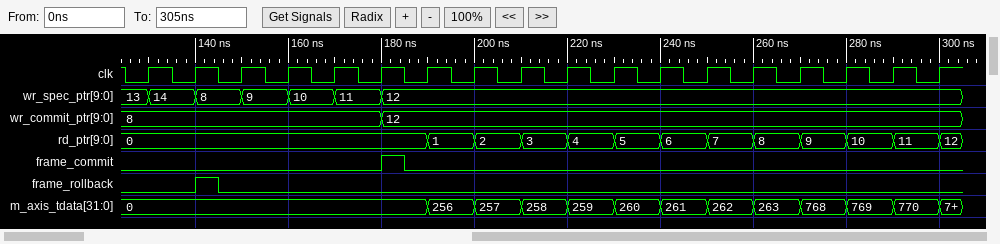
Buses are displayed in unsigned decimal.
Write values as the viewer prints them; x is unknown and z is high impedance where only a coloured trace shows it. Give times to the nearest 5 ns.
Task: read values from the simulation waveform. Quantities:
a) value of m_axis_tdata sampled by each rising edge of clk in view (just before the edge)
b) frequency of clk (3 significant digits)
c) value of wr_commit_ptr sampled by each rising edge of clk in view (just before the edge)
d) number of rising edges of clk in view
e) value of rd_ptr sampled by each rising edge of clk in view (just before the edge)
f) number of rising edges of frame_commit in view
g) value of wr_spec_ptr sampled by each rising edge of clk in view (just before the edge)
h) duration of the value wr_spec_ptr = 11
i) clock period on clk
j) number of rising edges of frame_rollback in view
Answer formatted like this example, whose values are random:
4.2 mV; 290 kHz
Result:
0, 0, 0, 0, 0, 0, 0, 256, 257, 258, 259, 260, 261, 262, 263, 768, 769, 770; 100 MHz; 8, 8, 8, 8, 8, 8, 12, 12, 12, 12, 12, 12, 12, 12, 12, 12, 12, 12; 18; 0, 0, 0, 0, 0, 0, 0, 1, 2, 3, 4, 5, 6, 7, 8, 9, 10, 11; 1; 13, 14, 8, 9, 10, 11, 12, 12, 12, 12, 12, 12, 12, 12, 12, 12, 12, 12; 10 ns; 10 ns; 1
